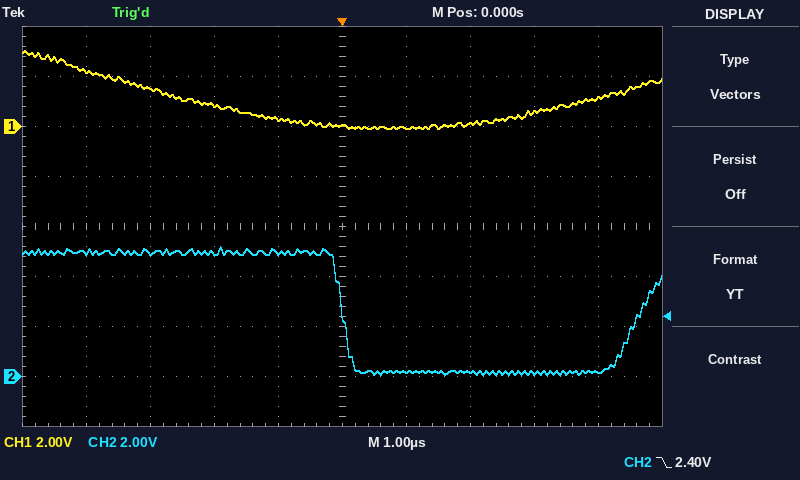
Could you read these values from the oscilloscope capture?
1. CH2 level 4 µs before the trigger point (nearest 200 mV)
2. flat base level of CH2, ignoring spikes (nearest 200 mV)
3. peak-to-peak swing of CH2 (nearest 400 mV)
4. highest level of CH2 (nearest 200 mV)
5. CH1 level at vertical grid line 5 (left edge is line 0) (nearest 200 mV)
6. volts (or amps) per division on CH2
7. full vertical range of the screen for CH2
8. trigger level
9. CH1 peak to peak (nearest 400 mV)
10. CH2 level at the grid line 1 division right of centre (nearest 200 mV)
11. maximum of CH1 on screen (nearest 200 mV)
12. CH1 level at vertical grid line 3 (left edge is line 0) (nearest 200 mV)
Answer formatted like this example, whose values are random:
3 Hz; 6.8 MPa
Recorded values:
5.0 V; 200 mV; 5.2 V; 5.2 V; 0.0 V; 2 V; 16 V; 2.40 V; 3.2 V; 200 mV; 3.0 V; 800 mV
